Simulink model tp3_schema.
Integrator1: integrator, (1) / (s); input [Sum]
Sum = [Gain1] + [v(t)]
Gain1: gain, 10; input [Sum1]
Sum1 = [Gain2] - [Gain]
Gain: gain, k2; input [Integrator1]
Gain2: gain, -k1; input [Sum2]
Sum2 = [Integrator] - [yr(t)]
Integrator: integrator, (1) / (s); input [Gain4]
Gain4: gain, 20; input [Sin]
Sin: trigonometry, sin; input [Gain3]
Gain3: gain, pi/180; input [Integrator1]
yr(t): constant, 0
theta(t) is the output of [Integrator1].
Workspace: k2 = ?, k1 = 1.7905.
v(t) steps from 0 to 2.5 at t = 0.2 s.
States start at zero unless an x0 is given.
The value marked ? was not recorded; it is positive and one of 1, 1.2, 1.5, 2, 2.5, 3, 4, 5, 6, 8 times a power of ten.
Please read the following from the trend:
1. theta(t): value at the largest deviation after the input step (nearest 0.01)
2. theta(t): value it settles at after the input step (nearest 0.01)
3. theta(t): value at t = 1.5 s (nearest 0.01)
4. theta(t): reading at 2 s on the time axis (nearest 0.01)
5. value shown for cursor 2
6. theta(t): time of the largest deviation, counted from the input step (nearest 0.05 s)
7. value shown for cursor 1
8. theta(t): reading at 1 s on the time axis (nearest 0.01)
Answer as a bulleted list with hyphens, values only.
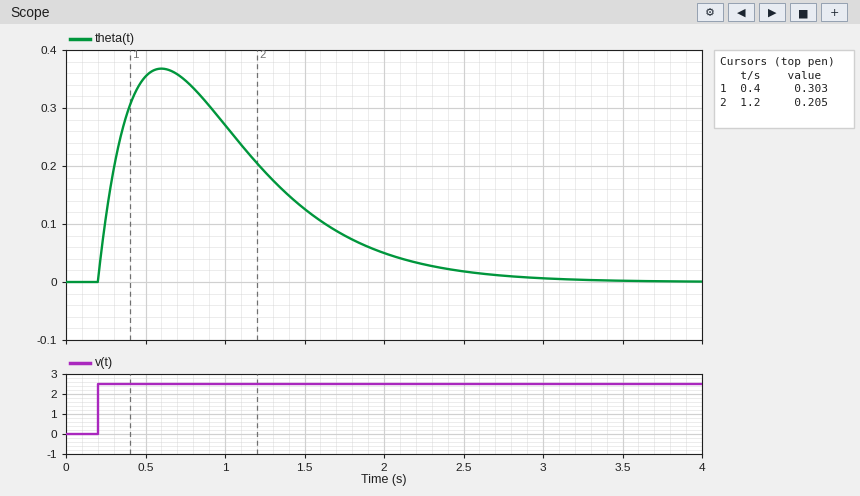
- 0.37
- 0.00
- 0.13
- 0.05
- 0.205
- 0.40 s
- 0.303
- 0.27
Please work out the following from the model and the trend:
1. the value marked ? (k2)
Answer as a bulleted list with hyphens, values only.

- 0.5
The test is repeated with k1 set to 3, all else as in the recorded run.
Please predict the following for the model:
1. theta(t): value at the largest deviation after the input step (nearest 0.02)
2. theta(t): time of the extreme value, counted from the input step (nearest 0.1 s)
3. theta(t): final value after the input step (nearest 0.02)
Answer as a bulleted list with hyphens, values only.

- 0.34
- 0.3 s
- 0.00
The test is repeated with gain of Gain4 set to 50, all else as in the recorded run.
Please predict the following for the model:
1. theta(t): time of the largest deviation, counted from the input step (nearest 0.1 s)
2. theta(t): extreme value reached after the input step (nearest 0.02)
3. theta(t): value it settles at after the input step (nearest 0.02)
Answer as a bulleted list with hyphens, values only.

- 0.3 s
- 0.30
- 0.00
